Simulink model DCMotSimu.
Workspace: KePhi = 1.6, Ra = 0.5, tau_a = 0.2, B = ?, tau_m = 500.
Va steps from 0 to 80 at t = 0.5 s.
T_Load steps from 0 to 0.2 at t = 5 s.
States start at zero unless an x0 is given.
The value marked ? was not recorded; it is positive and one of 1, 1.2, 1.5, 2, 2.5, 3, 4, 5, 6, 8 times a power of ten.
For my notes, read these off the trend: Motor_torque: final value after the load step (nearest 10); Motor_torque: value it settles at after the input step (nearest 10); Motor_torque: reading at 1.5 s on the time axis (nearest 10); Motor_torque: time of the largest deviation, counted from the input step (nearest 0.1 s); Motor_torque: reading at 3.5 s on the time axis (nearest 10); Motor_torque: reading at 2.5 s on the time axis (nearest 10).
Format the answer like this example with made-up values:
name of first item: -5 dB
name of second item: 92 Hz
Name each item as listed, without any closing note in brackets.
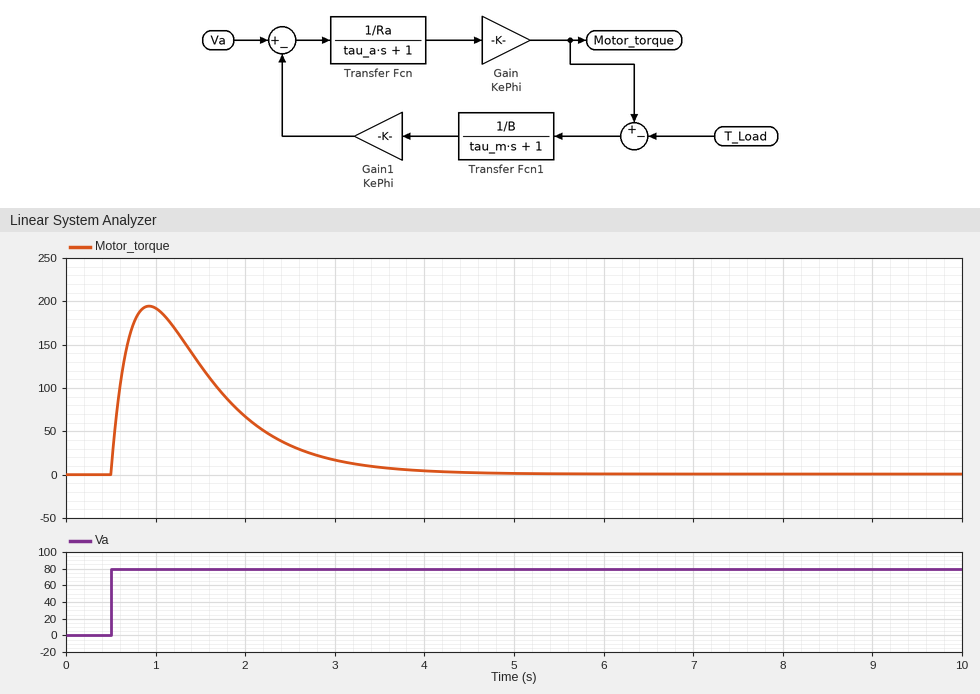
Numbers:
Motor_torque: final value after the load step: 0
Motor_torque: value it settles at after the input step: 0
Motor_torque: reading at 1.5 s on the time axis: 130
Motor_torque: time of the largest deviation, counted from the input step: 0.4 s
Motor_torque: reading at 3.5 s on the time axis: 10
Motor_torque: reading at 2.5 s on the time axis: 30
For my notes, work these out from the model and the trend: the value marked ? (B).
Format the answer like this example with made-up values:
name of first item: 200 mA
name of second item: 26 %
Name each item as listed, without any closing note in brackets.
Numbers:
the value marked ?: 0.01
